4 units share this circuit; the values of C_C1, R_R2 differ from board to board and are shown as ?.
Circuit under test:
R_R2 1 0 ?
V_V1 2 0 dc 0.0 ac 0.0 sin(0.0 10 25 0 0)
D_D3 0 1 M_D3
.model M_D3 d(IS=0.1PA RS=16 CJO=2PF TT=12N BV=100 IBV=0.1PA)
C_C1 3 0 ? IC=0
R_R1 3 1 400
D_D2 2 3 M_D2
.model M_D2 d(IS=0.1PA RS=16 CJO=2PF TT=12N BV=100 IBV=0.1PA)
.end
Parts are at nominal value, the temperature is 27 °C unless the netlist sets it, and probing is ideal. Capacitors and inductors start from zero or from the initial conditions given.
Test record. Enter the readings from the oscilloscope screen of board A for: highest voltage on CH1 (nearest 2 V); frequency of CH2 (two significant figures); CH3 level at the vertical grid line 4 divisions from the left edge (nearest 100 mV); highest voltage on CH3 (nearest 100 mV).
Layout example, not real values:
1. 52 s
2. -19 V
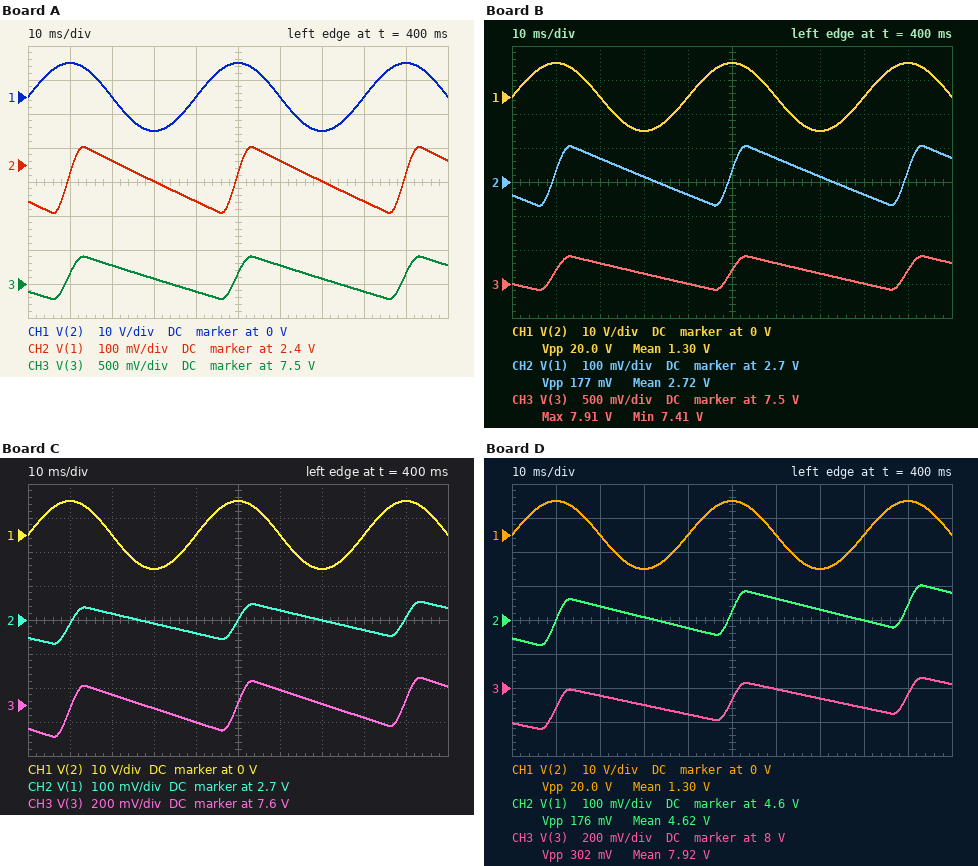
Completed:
1. 10 V
2. 25 Hz
3. 7.4 V
4. 7.9 V
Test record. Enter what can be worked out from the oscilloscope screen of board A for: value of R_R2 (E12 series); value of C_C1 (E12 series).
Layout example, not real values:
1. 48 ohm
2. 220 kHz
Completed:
1. 180 Ω
2. 680 µF
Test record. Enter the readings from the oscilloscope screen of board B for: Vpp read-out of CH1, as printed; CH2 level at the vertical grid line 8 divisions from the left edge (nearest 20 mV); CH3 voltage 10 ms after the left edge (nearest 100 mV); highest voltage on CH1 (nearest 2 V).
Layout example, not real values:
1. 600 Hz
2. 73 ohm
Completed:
1. 20.0 V
2. 2.66 V
3. 7.7 V
4. 10 V
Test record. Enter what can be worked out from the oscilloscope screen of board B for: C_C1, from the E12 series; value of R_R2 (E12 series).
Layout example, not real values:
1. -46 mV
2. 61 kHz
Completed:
1. 820 µF
2. 220 Ω
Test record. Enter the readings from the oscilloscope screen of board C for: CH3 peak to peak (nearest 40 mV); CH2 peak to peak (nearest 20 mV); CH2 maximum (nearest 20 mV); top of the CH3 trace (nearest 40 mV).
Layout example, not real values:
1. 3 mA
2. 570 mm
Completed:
1. 360 mV
2. 120 mV
3. 2.76 V
4. 7.76 V
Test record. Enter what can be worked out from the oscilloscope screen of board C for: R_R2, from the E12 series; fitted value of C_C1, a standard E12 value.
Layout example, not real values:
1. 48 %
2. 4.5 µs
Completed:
1. 220 Ω
2. 1.5 mF
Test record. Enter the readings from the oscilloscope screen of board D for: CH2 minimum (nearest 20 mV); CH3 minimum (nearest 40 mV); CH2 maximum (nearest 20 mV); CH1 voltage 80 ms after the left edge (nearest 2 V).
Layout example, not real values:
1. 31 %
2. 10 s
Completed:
1. 4.52 V
2. 7.76 V
3. 4.70 V
4. 0 V
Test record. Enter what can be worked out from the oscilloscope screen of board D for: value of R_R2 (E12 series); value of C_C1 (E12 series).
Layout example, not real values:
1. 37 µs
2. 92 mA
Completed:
1. 560 Ω
2. 1.5 mF
